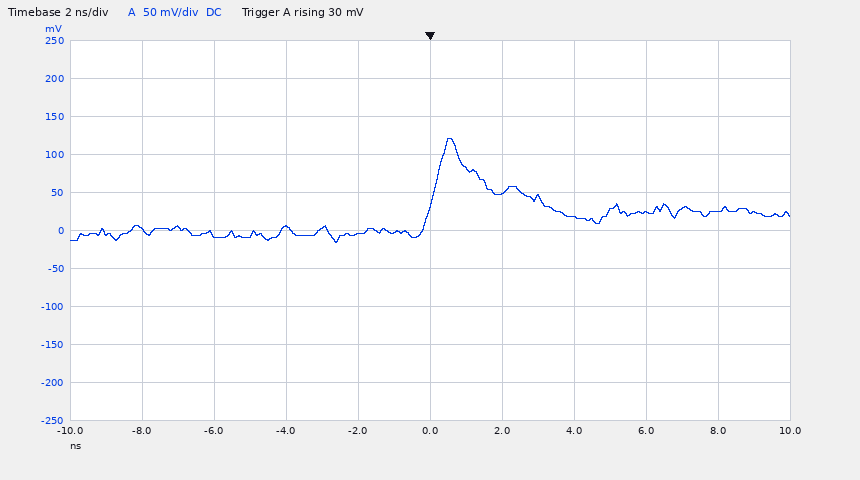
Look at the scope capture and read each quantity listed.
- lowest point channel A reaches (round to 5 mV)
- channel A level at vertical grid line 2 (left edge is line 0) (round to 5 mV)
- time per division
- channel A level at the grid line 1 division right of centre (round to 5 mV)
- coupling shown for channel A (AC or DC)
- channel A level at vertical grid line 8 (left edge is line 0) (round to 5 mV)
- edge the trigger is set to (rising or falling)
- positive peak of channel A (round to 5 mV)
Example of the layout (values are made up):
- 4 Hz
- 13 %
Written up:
- -15 mV
- -5 mV
- 2 ns
- 50 mV
- DC
- 25 mV
- rising
- 120 mV
